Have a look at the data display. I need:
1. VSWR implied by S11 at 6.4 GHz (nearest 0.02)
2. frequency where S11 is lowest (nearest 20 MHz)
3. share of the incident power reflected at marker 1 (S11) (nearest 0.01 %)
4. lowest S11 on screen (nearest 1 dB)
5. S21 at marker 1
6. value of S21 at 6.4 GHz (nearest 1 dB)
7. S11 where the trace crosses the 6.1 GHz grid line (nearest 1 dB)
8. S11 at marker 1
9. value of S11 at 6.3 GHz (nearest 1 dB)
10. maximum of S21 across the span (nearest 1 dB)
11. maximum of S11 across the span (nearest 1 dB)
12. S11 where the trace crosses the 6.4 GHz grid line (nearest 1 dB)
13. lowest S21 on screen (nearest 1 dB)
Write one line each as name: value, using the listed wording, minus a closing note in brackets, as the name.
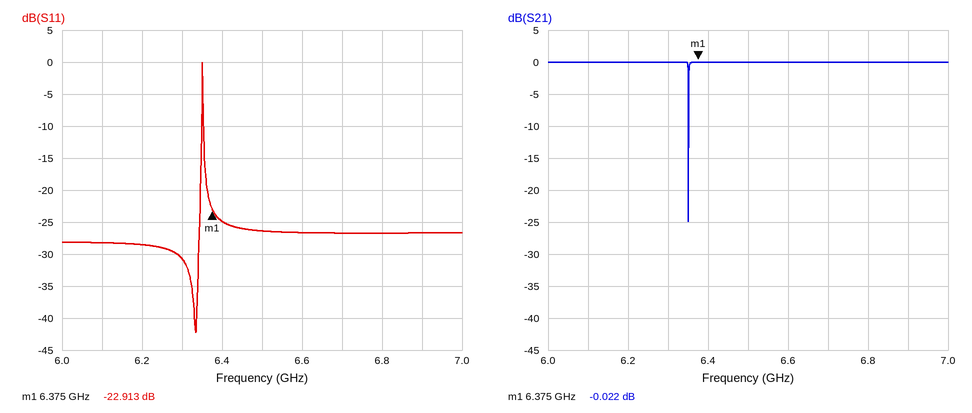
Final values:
VSWR implied by S11 at 6.4 GHz: 1.12
frequency where S11 is lowest: 6.34 GHz
share of the incident power reflected at marker 1 (S11): 0.51 %
lowest S11 on screen: -42 dB
S21 at marker 1: -0.022 dB
value of S21 at 6.4 GHz: 0 dB
S11 where the trace crosses the 6.1 GHz grid line: -28 dB
S11 at marker 1: -22.913 dB
value of S11 at 6.3 GHz: -31 dB
maximum of S21 across the span: 0 dB
maximum of S11 across the span: 0 dB
S11 where the trace crosses the 6.4 GHz grid line: -25 dB
lowest S21 on screen: -25 dB
